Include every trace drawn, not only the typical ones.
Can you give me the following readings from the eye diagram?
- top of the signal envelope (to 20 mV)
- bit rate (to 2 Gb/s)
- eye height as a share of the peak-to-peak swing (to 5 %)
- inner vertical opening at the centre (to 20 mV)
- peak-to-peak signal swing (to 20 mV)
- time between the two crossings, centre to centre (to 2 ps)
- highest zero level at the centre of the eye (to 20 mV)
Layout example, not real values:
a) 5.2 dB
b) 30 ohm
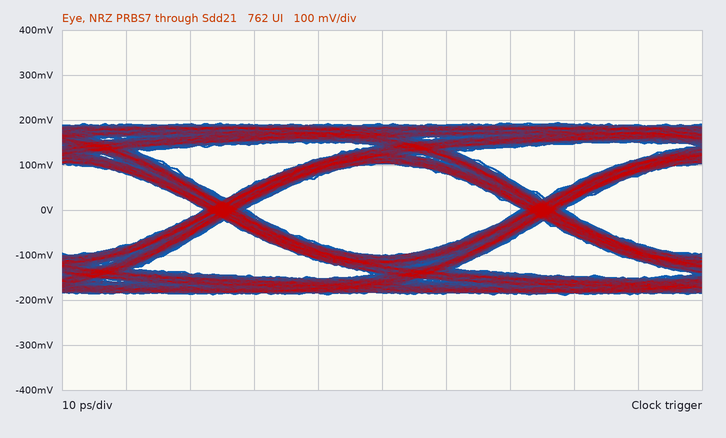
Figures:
a) 200 mV
b) 20 Gb/s
c) 55 %
d) 200 mV
e) 380 mV
f) 50 ps
g) -100 mV
